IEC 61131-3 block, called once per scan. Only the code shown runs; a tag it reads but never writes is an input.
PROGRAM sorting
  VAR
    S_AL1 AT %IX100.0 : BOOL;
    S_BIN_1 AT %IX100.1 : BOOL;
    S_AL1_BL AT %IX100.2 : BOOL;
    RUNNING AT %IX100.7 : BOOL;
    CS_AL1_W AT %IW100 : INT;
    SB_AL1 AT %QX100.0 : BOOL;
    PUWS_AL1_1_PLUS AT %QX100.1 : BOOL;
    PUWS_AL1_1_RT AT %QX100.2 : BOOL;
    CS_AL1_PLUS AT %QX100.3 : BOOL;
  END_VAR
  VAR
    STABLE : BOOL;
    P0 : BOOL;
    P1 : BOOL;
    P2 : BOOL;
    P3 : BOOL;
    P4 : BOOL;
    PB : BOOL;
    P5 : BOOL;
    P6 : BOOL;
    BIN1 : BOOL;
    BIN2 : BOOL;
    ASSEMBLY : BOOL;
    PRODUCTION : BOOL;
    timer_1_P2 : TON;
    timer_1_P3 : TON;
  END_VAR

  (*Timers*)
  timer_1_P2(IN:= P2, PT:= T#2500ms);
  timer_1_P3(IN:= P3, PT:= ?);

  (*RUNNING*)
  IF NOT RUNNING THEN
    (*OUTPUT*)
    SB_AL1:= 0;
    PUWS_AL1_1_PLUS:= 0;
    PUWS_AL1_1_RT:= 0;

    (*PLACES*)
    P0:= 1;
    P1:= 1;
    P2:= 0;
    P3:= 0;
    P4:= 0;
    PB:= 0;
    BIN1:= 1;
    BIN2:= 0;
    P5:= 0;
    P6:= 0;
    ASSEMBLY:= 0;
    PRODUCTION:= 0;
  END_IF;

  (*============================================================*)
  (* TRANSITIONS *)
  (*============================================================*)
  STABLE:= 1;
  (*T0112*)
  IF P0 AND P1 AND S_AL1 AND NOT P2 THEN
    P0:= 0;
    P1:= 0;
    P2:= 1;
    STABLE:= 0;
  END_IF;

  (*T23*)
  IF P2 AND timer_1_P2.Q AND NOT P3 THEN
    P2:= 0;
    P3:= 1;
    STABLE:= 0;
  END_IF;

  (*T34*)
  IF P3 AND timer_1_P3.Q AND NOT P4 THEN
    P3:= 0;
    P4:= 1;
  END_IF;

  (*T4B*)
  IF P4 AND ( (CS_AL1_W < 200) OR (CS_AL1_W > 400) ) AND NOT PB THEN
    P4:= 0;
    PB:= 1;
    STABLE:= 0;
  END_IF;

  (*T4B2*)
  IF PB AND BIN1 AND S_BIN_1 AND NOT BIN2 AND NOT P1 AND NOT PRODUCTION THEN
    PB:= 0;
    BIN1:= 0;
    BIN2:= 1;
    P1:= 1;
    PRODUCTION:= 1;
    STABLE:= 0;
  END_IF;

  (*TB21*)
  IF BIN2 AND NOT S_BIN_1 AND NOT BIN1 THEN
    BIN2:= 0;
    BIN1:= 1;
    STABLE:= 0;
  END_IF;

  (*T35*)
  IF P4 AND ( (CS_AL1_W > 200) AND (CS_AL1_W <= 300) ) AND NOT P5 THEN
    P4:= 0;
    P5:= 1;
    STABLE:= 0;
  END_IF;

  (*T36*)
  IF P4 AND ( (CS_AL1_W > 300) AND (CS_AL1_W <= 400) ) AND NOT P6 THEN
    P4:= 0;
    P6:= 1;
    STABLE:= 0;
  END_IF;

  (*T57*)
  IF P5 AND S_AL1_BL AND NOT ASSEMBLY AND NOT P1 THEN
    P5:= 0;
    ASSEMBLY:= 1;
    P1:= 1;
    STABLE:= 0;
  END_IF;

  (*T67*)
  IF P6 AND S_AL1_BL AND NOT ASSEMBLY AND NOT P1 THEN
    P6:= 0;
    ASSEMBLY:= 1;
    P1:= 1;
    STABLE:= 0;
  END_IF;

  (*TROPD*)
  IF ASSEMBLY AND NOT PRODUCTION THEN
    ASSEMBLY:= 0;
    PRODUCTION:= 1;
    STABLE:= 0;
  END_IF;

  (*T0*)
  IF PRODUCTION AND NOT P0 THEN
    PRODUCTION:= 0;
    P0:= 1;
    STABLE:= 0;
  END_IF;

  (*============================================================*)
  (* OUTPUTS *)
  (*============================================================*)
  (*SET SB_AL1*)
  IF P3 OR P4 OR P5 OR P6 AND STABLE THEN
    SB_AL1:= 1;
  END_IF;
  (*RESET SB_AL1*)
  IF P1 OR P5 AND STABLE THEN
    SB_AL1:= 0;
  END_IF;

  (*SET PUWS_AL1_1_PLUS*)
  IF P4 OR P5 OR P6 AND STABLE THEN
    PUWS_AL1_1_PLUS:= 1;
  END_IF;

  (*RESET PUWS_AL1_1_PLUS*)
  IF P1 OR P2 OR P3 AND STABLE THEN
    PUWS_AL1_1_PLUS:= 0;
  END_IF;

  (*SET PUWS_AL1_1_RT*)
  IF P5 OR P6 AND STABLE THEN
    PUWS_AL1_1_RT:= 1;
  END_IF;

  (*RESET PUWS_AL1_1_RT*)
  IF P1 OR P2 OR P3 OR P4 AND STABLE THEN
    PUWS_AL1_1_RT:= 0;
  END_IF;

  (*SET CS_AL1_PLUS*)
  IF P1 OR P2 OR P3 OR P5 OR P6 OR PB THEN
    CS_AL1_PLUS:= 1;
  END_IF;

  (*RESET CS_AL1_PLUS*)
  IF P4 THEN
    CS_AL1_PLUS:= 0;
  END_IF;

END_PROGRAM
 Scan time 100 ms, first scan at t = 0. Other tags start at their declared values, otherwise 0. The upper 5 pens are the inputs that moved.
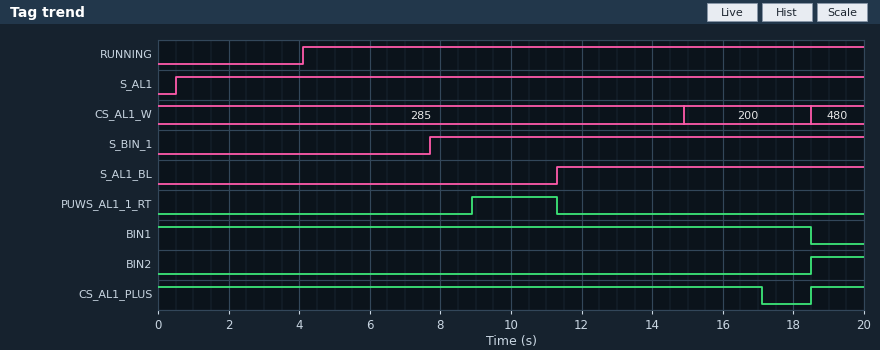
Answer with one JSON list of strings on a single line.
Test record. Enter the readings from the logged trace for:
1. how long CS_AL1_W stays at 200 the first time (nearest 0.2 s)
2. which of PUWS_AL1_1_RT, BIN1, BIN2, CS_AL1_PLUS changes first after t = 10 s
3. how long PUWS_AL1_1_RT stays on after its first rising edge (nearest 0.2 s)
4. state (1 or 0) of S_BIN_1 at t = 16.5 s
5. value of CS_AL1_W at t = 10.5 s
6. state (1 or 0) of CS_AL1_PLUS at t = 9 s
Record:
["3.6 s", "PUWS_AL1_1_RT", "2.4 s", "1", "285", "1"]
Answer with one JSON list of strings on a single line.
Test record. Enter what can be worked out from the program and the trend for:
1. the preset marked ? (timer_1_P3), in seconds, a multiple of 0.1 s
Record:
["3.0 s"]
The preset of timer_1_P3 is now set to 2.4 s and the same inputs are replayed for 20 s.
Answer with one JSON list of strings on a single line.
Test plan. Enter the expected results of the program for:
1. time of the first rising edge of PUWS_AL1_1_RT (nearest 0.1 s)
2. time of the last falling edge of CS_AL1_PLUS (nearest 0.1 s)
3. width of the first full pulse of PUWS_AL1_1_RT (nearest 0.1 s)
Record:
["8.3 s", "16.5 s", "3.0 s"]
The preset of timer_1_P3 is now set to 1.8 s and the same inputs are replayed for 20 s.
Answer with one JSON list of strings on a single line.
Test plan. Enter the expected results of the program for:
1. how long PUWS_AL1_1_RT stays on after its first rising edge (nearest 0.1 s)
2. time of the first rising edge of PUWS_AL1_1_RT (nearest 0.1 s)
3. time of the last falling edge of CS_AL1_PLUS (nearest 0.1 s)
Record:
["3.6 s", "7.7 s", "15.9 s"]
